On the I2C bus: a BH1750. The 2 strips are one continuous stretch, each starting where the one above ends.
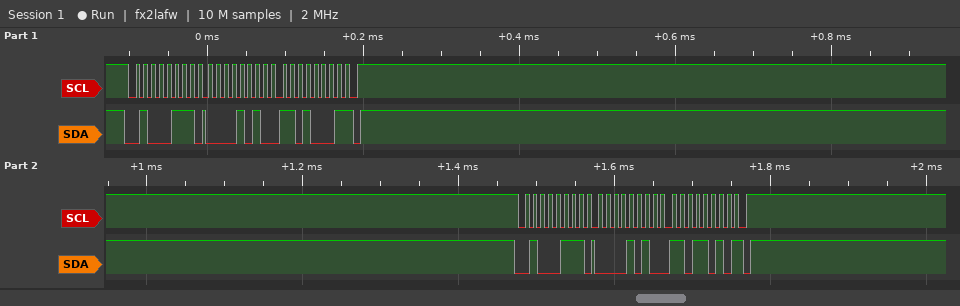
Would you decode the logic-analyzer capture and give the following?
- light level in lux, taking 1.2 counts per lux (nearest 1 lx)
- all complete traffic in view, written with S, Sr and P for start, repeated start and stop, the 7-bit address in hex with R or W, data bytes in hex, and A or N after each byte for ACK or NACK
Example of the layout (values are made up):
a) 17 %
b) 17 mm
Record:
a) 2308 lx
b) S 23R A 0A A D1 N P S 23R A 0A A DA N P
